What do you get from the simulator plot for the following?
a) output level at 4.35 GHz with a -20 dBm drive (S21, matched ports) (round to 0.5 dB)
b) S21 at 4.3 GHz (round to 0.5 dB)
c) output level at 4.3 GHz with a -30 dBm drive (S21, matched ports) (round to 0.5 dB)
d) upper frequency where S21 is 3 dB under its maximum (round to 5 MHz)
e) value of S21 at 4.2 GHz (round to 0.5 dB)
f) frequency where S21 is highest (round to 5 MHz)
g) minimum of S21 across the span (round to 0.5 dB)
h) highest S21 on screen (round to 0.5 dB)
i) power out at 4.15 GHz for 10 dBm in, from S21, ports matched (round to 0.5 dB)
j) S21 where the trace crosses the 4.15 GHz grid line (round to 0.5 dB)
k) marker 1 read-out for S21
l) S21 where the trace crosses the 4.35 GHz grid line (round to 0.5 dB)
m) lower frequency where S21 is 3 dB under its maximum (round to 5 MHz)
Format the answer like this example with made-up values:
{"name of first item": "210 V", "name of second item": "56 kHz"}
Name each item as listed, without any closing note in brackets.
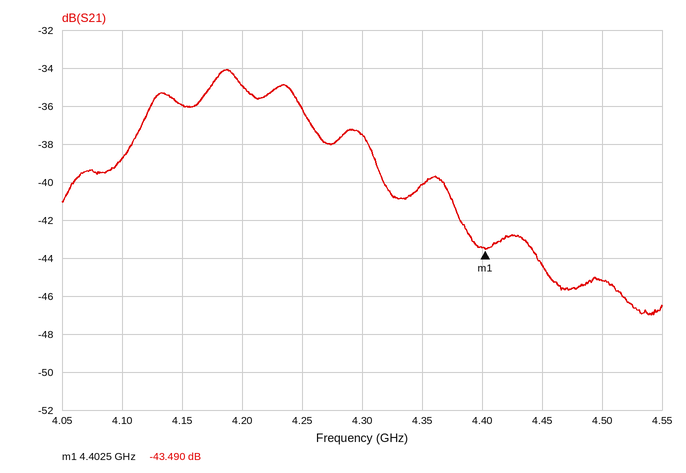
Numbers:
{"output level at 4.35 GHz with a -20 dBm drive (S21, matched ports)": "-60.0 dBm", "S21 at 4.3 GHz": "-37.5 dB", "output level at 4.3 GHz with a -30 dBm drive (S21, matched ports)": "-67.5 dBm", "upper frequency where S21 is 3 dB under its maximum": "4.260 GHz", "value of S21 at 4.2 GHz": "-35.0 dB", "frequency where S21 is highest": "4.185 GHz", "minimum of S21 across the span": "-47.0 dB", "highest S21 on screen": "-34.0 dB", "power out at 4.15 GHz for 10 dBm in, from S21, ports matched": "-26.0 dBm", "S21 where the trace crosses the 4.15 GHz grid line": "-36.0 dB", "marker 1 read-out for S21": "-43.490 dB", "S21 where the trace crosses the 4.35 GHz grid line": "-40.0 dB", "lower frequency where S21 is 3 dB under its maximum": "4.115 GHz"}
